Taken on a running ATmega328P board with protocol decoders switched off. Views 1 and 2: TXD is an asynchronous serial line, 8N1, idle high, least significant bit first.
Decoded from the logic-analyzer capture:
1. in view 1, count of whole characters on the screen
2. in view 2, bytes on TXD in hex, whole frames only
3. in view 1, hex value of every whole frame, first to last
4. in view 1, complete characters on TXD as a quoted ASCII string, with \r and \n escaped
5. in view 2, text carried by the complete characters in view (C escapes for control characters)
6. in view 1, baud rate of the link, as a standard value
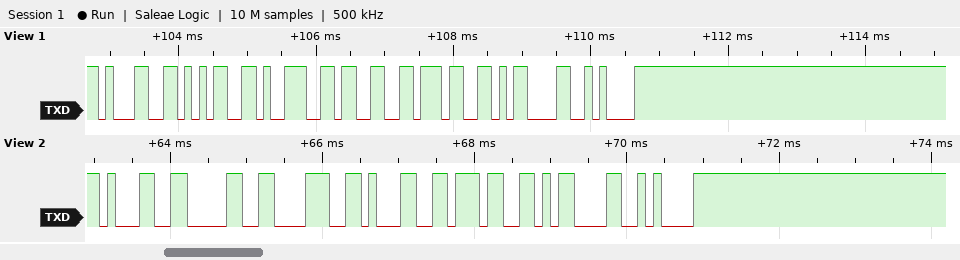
7
31 30 38 31 37 0D 0A
0x31 0x35 0x39 0x33 0x37 0x0D 0x0A
"15937\r\n"
"10817\r\n"
9600 baud
